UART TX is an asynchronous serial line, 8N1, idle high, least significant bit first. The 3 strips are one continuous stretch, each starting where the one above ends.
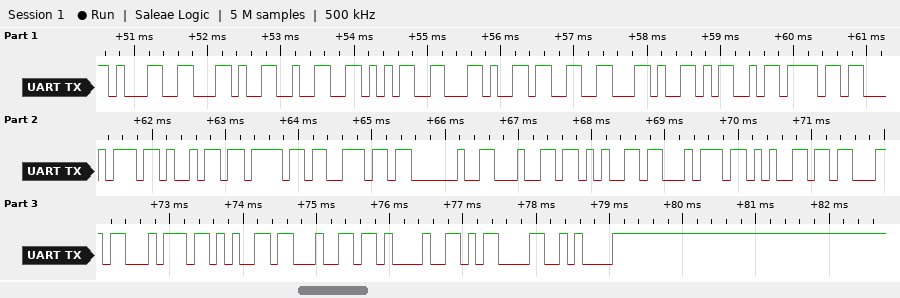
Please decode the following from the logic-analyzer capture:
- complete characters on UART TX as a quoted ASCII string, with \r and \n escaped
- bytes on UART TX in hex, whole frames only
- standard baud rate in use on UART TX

"1,25,3,Motion detected!\r\n"
31 2C 32 35 2C 33 2C 4D 6F 74 69 6F 6E 20 64 65 74 65 63 74 65 64 21 0D 0A
9600 baud
